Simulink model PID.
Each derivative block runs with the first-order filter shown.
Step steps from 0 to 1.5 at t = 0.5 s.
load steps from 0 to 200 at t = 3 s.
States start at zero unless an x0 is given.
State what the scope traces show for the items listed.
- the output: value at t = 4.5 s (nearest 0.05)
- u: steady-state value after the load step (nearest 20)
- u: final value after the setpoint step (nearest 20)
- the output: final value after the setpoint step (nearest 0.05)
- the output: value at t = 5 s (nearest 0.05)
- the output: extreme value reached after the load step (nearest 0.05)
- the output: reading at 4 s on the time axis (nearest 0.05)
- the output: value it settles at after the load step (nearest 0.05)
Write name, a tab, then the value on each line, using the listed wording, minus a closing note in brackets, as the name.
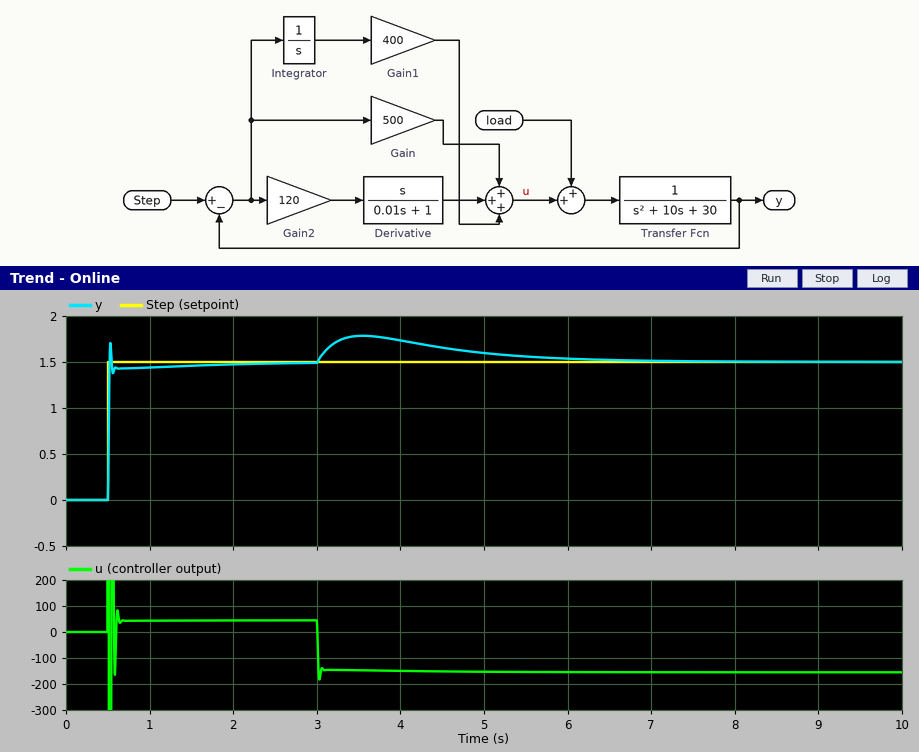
the output: value at t = 4.5 s	1.65
u: steady-state value after the load step	-160
u: final value after the setpoint step	40
the output: final value after the setpoint step	1.50
the output: value at t = 5 s	1.60
the output: extreme value reached after the load step	1.80
the output: reading at 4 s on the time axis	1.75
the output: value it settles at after the load step	1.50
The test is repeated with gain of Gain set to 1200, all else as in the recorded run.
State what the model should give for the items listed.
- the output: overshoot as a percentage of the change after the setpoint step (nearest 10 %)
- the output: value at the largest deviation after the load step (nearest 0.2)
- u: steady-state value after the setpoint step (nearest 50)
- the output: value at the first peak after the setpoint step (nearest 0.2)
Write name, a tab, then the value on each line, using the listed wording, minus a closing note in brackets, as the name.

the output: overshoot as a percentage of the change after the setpoint step	20 %
the output: value at the largest deviation after the load step	1.6
u: steady-state value after the setpoint step	50
the output: value at the first peak after the setpoint step	1.8
